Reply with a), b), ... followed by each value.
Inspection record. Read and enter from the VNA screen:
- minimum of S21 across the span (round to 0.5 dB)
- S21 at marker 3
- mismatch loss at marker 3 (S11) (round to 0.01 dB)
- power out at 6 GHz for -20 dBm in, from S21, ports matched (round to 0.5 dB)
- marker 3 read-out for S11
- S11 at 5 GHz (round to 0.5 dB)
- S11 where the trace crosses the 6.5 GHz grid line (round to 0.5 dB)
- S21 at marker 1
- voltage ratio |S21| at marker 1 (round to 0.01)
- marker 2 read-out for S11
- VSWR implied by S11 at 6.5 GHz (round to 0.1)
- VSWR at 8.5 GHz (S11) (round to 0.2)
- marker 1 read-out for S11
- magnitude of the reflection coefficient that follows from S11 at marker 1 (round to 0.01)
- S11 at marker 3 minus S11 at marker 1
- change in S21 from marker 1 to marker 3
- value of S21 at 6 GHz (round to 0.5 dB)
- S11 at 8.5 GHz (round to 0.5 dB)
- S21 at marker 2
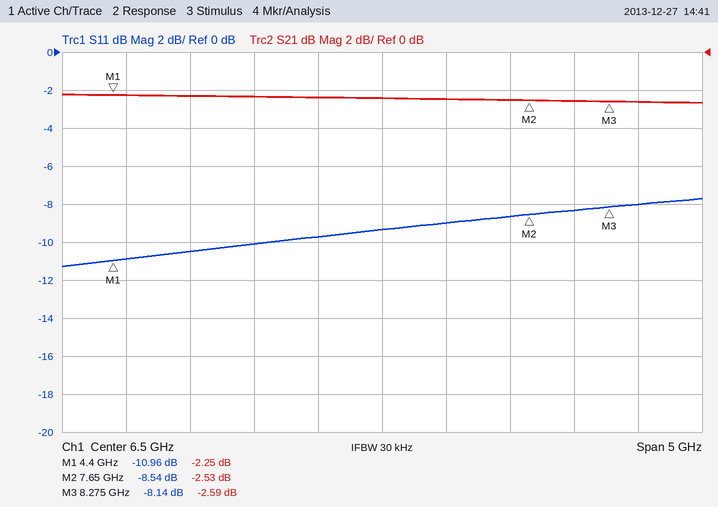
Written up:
a) -2.5 dB
b) -2.59 dB
c) 0.72 dB
d) -22.5 dBm
e) -8.14 dB
f) -10.5 dB
g) -9.5 dB
h) -2.25 dB
i) 0.77
j) -8.54 dB
k) 2.0
l) 2.4
m) -10.96 dB
n) 0.28
o) 2.82 dB
p) -0.34 dB
q) -2.5 dB
r) -8.0 dB
s) -2.53 dB
